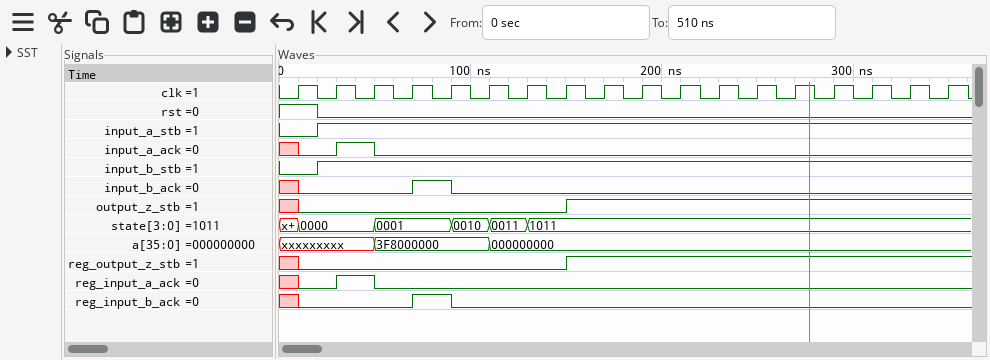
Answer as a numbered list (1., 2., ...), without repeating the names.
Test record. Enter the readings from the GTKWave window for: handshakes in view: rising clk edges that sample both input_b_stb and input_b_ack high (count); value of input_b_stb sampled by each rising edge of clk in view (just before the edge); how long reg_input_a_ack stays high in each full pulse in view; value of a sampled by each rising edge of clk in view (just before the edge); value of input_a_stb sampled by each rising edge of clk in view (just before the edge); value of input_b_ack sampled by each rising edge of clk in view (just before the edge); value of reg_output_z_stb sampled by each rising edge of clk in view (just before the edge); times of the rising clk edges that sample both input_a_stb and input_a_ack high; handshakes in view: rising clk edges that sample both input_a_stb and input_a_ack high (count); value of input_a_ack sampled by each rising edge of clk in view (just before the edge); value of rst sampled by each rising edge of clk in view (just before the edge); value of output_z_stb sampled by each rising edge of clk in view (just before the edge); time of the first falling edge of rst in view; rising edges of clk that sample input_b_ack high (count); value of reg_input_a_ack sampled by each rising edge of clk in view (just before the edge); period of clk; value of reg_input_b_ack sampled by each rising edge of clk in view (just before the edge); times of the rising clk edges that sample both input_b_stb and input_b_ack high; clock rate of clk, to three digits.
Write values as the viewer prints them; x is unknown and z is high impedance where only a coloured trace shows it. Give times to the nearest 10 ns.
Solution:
1. 1
2. 0 1 1 1 1 1 1 1 1 1 1 1 1 1 1 1 1 1
3. 20 ns
4. xxxxxxxxx, xxxxxxxxx, xxxxxxxxx, 3F8000000, 3F8000000, 3F8000000, 000000000, 000000000, 000000000, 000000000, 000000000, 000000000, 000000000, 000000000, 000000000, 000000000, 000000000, 000000000
5. 0 1 1 1 1 1 1 1 1 1 1 1 1 1 1 1 1 1
6. x 0 0 0 1 0 0 0 0 0 0 0 0 0 0 0 0 0
7. x 0 0 0 0 0 0 0 1 1 1 1 1 1 1 1 1 1
8. 50 ns
9. 1
10. x 0 1 0 0 0 0 0 0 0 0 0 0 0 0 0 0 0
11. 1 0 0 0 0 0 0 0 0 0 0 0 0 0 0 0 0 0
12. x 0 0 0 0 0 0 0 1 1 1 1 1 1 1 1 1 1
13. 20 ns
14. 1
15. x 0 1 0 0 0 0 0 0 0 0 0 0 0 0 0 0 0
16. 20 ns
17. x 0 0 0 1 0 0 0 0 0 0 0 0 0 0 0 0 0
18. 90 ns
19. 50.0 MHz
